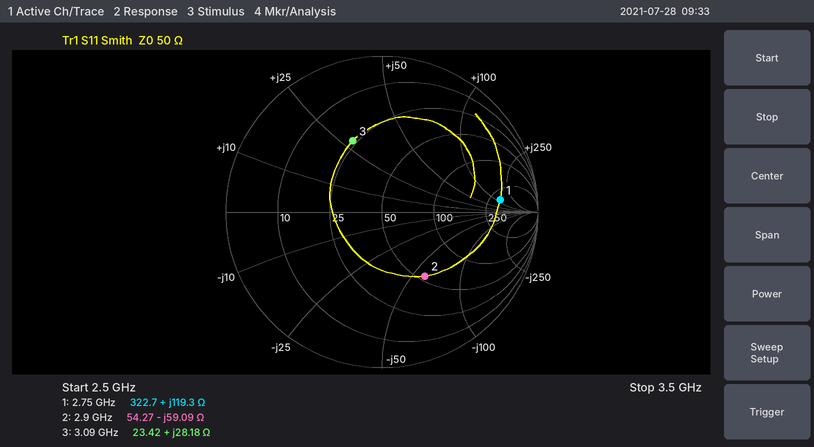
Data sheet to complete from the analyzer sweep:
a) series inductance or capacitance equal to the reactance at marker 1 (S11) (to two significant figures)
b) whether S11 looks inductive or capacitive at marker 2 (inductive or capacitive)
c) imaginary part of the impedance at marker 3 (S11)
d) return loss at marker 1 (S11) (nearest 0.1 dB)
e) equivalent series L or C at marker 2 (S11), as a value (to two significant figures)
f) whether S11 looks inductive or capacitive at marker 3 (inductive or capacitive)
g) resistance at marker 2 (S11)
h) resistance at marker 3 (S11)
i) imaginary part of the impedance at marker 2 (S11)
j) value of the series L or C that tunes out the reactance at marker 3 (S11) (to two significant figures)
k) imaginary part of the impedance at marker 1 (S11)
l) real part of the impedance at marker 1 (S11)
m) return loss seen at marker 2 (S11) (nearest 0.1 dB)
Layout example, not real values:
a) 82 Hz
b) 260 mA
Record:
a) 6.9 nH
b) capacitive
c) +28.18 Ω
d) 2.4 dB
e) 930 fF
f) inductive
g) 54.27 Ω
h) 23.42 Ω
i) -59.09 Ω
j) 1.8 pF
k) +119.3 Ω
l) 322.7 Ω
m) 6.1 dB
